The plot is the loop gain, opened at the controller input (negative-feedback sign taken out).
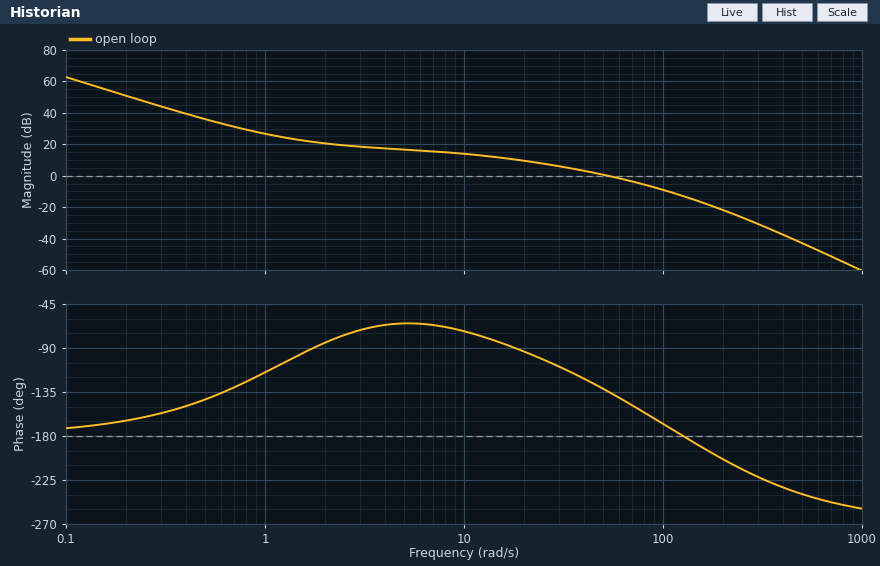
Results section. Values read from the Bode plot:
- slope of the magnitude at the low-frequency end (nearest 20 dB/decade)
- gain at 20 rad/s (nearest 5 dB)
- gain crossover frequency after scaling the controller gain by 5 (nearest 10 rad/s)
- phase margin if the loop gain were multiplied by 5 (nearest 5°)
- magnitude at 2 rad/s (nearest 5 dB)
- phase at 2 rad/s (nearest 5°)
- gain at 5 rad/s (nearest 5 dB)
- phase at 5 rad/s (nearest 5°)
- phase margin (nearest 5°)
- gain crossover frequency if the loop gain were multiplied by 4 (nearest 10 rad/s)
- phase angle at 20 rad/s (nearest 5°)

-40 dB/decade
10 dB
130 rad/s
-5°
20 dB
-85°
15 dB
-65°
45°
120 rad/s
-95°
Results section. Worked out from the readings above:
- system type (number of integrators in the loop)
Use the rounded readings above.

2
